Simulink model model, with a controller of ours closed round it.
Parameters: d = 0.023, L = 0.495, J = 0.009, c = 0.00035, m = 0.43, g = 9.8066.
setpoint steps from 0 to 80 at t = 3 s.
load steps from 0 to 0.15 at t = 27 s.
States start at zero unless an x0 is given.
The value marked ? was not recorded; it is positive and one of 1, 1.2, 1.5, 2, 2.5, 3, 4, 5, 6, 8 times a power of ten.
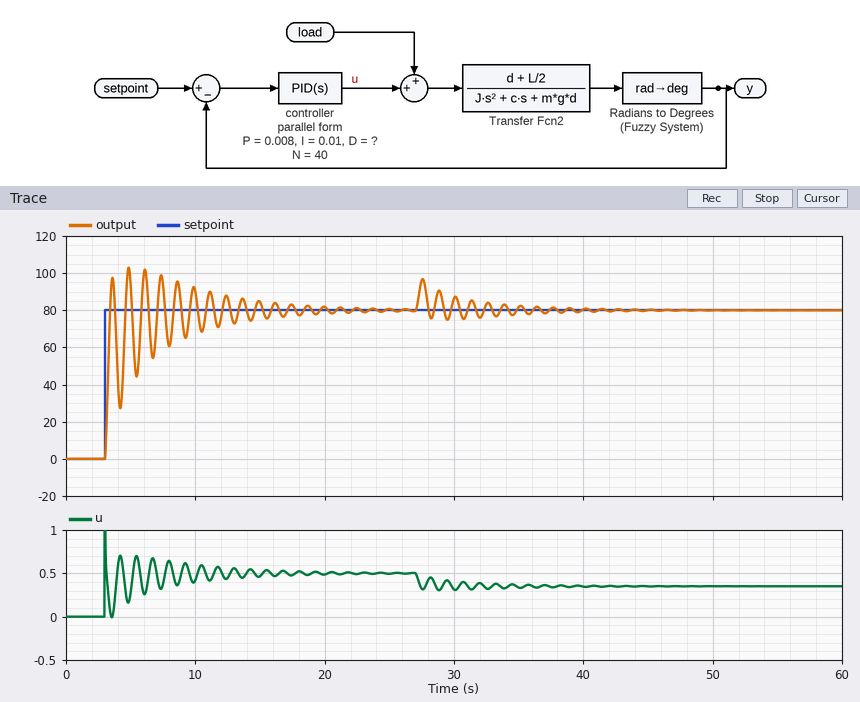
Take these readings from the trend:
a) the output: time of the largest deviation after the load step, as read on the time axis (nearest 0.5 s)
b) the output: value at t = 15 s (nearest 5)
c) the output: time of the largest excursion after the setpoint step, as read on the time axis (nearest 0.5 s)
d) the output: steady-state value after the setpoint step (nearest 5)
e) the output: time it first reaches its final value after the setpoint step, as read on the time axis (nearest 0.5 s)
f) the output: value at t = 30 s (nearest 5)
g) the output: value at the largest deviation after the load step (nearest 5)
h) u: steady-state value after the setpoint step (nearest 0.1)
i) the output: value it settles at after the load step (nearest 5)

27.5 s
85
5.0 s
80
3.5 s
85
95
0.5
80
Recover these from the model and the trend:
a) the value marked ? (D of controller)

0.0006
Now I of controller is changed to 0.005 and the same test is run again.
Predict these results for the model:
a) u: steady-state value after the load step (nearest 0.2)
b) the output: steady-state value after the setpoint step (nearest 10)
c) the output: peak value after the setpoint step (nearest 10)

0.4
80
90
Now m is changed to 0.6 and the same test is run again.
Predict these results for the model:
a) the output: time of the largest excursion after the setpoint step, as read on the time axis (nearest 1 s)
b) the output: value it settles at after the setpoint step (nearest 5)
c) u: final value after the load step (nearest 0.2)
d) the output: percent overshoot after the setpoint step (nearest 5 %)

6 s
80
0.6
15 %
